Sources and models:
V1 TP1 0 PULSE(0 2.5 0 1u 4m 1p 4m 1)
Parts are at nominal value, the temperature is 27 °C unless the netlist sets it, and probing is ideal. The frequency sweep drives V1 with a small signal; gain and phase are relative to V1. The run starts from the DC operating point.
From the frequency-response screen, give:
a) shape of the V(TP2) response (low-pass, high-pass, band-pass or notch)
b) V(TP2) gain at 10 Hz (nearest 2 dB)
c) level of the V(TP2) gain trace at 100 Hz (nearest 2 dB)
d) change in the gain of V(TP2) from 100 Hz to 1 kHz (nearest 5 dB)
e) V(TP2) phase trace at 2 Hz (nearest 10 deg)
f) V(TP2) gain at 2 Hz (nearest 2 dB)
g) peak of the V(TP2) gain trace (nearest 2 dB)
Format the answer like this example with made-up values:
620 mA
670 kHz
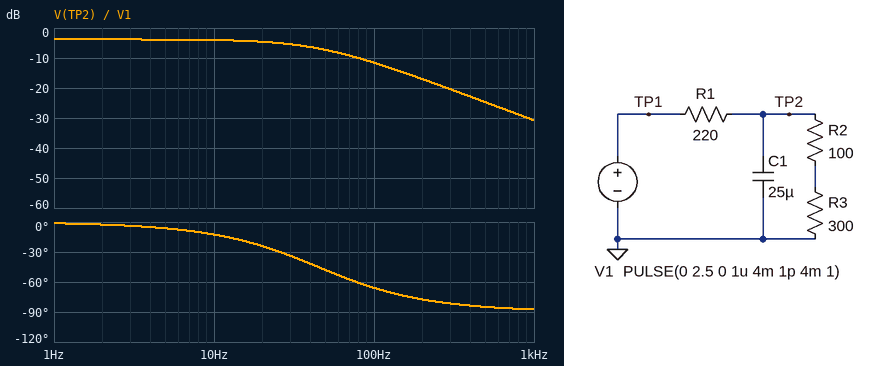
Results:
low-pass
-4 dB
-12 dB
-20 dB
0 deg
-4 dB
-4 dB
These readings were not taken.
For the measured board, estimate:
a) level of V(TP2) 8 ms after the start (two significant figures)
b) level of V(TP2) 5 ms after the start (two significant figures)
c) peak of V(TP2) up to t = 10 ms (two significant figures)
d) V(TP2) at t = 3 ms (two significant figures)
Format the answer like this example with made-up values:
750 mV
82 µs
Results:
140 mV
340 mV
530 mV
530 mV
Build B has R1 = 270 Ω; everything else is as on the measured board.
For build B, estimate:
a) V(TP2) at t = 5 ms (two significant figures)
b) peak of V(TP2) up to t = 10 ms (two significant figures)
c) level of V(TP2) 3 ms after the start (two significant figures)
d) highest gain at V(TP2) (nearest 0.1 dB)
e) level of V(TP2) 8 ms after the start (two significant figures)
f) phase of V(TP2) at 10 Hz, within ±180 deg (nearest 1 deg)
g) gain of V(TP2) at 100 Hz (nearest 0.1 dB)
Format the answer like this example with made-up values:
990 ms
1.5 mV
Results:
310 mV
460 mV
450 mV
-4.5 dB
150 mV
-14 deg
-13.2 dB
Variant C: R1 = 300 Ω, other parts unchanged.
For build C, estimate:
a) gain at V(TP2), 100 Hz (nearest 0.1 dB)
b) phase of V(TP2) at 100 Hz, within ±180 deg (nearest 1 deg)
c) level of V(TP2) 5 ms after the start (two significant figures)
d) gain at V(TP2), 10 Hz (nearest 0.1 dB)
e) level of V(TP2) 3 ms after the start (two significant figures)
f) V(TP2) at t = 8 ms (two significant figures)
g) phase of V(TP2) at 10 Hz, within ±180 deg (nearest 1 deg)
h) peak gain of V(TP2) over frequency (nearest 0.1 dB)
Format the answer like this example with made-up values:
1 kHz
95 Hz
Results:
-14.0 dB
-70 deg
290 mV
-5.2 dB
420 mV
140 mV
-15 deg
-4.9 dB
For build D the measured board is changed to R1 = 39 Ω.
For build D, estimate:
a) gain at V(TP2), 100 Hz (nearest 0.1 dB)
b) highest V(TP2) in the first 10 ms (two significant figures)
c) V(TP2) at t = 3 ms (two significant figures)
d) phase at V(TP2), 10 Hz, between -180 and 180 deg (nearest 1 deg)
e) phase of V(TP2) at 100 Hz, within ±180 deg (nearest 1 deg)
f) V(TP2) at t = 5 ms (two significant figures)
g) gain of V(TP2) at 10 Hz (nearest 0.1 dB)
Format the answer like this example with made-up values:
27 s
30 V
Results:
-2.0 dB
1.4 V
980 mV
-3 deg
-29 deg
150 mV
-0.8 dB
